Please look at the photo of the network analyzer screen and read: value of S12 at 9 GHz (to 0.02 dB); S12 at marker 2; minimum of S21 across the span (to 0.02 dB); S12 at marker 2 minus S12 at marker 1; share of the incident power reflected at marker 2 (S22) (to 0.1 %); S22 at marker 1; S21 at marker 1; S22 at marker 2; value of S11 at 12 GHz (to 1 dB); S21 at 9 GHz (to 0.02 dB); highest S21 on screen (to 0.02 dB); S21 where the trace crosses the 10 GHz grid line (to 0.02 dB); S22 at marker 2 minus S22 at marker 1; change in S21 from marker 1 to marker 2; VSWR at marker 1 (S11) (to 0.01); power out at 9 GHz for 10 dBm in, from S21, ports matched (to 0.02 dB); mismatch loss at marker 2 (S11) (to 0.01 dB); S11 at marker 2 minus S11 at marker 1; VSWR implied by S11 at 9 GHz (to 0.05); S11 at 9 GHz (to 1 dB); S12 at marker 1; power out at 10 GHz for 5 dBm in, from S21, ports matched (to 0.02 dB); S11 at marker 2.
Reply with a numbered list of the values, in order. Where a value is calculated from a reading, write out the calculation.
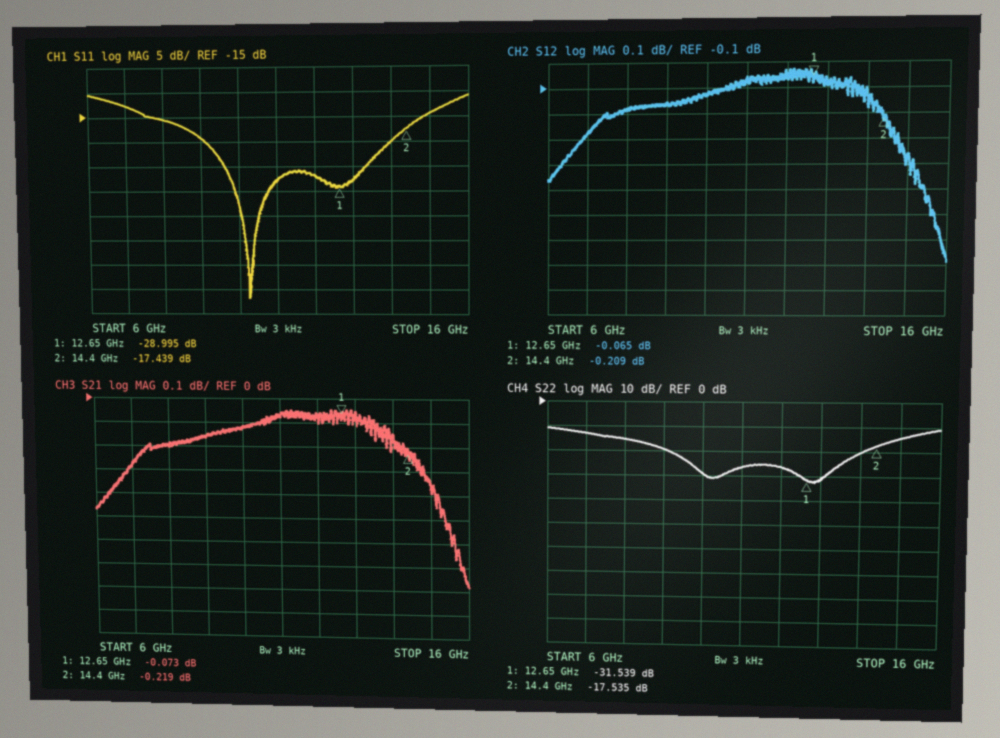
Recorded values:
1. -0.16 dB
2. -0.209 dB
3. -0.78 dB
4. -0.209 − (-0.065) = -0.144 dB
5. 10^(-17.535/10) ≈ 1.8 %
6. -31.539 dB
7. -0.073 dB
8. -17.535 dB
9. -27 dB
10. -0.16 dB
11. -0.04 dB
12. -0.12 dB
13. -17.535 − (-31.539) = 14.004 dB
14. -0.219 − (-0.073) = -0.146 dB
15. (1 + 0.0355)/(1 − 0.0355) ≈ 1.07
16. 10 dBm + (-0.16 dB) = 9.84 dBm
17. −10 log10(1 − 10^(-17.439/10)) ≈ 0.08 dB
18. -17.439 − (-28.995) = 11.556 dB
19. |Γ| = 10^(-19/20) = 0.1122; VSWR = (1 + 0.1122)/(1 − 0.1122) ≈ 1.25
20. -19 dB
21. -0.065 dB
22. 5 dBm + (-0.12 dB) = 4.88 dBm
23. -17.439 dB
